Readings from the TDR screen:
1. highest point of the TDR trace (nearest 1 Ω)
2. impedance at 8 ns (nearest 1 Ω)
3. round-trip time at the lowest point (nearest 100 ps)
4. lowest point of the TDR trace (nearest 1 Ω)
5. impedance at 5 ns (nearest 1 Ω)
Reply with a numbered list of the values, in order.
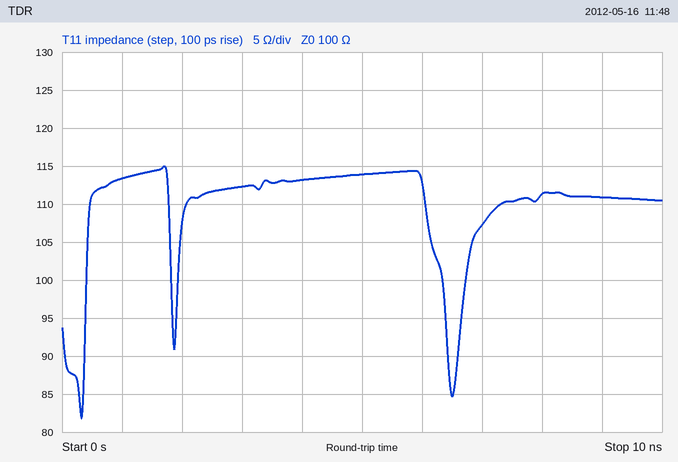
1. 115 Ω
2. 111 Ω
3. 300 ps
4. 82 Ω
5. 114 Ω
